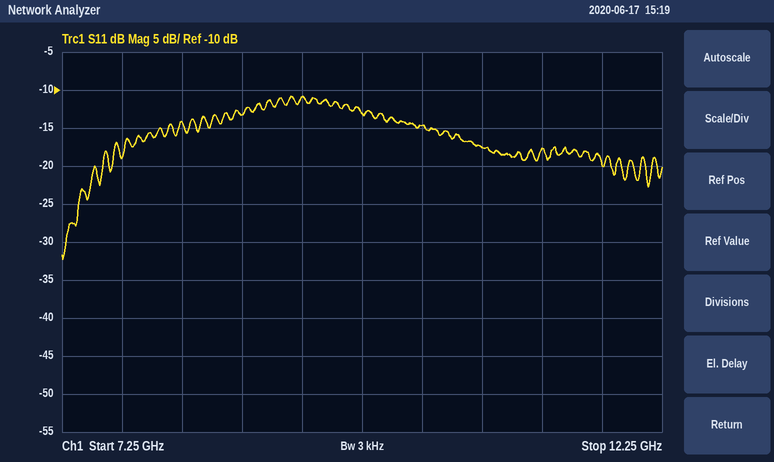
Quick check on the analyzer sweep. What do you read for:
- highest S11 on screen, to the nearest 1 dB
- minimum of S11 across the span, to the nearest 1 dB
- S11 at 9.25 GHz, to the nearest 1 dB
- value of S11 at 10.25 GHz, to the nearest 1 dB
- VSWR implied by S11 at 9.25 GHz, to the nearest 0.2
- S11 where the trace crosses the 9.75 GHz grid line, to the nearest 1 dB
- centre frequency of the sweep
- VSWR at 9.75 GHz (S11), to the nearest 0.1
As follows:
-11 dB
-32 dB
-11 dB
-15 dB
1.8
-13 dB
9.75 GHz
1.6
